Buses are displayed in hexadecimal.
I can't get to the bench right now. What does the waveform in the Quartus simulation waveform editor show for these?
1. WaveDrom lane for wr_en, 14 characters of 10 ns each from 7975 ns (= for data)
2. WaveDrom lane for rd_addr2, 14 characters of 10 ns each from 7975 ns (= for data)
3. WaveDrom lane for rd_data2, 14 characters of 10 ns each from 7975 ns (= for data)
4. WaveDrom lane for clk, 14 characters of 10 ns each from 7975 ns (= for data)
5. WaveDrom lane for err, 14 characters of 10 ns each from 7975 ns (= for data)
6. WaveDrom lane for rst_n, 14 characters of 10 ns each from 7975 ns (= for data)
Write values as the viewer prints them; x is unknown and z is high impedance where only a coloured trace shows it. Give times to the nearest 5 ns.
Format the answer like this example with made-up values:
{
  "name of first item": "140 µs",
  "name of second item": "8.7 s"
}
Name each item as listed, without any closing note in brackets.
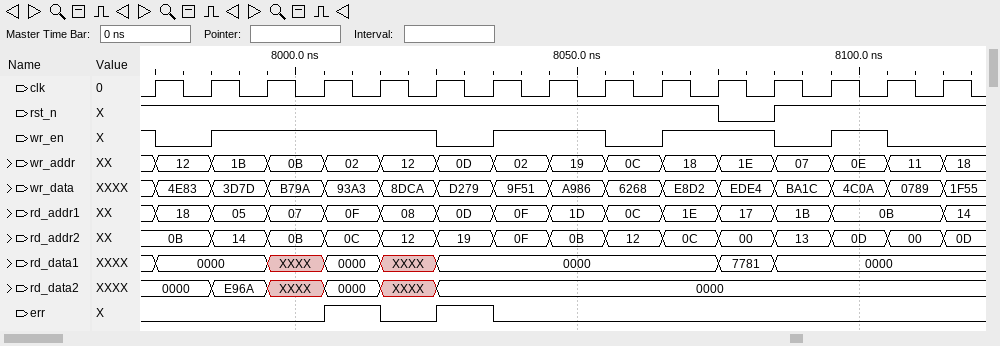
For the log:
{
  "WaveDrom lane for wr_en, 14 characters of 10 ns each from 7975 ns": "{name: 'wr_en', wave: '01...01.01.010'}",
  "WaveDrom lane for rd_addr2, 14 characters of 10 ns each from 7975 ns": "{name: 'rd_addr2', wave: '==============', data: '0B 14 0B 0C 12 19 0F 0B 12 0C 00 13 0D 00'}",
  "WaveDrom lane for rd_data2, 14 characters of 10 ns each from 7975 ns": "{name: 'rd_data2', wave: '==x=x=........', data: '0000 E96A 0000 0000'}",
  "WaveDrom lane for clk, 14 characters of 10 ns each from 7975 ns": "{name: 'clk', wave: 'p.............'}",
  "WaveDrom lane for err, 14 characters of 10 ns each from 7975 ns": "{name: 'err', wave: '0..1010.......'}",
  "WaveDrom lane for rst_n, 14 characters of 10 ns each from 7975 ns": "{name: 'rst_n', wave: '1.........01..'}"
}
